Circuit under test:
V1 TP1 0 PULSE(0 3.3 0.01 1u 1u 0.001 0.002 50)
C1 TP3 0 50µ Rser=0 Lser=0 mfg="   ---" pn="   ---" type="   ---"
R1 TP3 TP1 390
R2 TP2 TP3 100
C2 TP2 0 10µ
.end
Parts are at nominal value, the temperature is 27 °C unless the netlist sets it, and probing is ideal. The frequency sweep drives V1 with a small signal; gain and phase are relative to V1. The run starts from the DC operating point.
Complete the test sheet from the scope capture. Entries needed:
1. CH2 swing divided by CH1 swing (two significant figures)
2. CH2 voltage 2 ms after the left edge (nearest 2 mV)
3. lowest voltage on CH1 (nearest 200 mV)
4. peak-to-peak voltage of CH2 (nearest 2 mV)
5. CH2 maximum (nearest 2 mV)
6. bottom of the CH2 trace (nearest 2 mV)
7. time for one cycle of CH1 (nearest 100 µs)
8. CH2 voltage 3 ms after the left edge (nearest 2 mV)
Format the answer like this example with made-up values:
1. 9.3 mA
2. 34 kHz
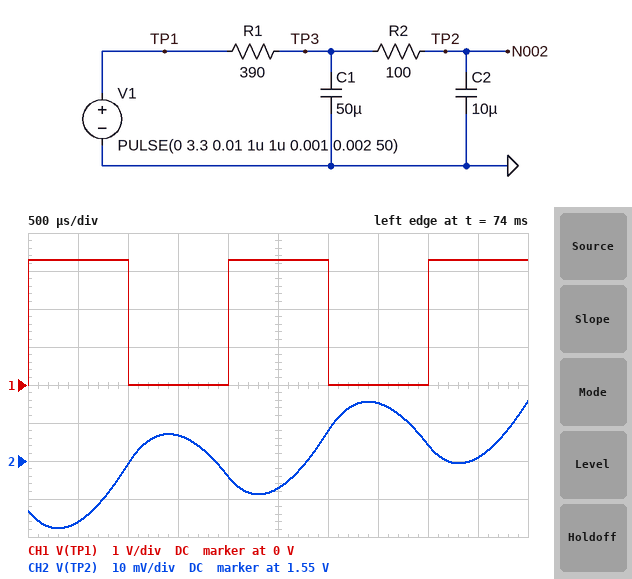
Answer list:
1. 0.010
2. 1.546 V
3. 0 V
4. 34 mV
5. 1.566 V
6. 1.532 V
7. 2.0 ms
8. 1.558 V
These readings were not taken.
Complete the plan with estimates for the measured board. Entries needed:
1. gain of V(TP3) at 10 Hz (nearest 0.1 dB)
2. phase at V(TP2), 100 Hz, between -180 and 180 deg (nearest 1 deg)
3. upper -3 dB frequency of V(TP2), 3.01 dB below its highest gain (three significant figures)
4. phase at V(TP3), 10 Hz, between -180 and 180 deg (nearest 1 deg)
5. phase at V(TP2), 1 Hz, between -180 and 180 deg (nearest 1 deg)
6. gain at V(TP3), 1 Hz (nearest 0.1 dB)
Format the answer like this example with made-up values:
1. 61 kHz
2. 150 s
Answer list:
1. -5.0 dB
2. -114 deg
3. 6.74 Hz
4. -55 deg
5. -9 deg
6. -0.1 dB
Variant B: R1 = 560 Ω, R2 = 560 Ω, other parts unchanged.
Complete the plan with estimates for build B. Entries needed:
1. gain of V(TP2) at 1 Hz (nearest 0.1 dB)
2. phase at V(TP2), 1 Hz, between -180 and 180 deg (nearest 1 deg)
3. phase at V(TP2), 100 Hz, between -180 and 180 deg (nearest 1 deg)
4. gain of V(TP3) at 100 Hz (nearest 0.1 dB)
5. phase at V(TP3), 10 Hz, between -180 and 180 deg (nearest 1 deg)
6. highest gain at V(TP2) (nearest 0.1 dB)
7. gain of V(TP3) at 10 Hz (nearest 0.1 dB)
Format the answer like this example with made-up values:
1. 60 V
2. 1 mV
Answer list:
1. -0.2 dB
2. -14 deg
3. -158 deg
4. -25.1 dB
5. -62 deg
6. 0 dB
7. -7.4 dB
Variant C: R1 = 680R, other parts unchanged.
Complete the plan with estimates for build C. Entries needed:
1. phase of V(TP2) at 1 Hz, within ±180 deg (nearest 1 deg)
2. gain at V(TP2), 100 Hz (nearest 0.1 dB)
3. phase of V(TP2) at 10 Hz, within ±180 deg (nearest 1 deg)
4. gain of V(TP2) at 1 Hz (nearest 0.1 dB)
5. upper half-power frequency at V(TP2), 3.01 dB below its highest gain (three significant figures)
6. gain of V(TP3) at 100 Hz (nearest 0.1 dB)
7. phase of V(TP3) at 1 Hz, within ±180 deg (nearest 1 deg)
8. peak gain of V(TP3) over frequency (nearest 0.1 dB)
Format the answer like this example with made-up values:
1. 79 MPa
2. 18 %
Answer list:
1. -15 deg
2. -29.3 dB
3. -72 deg
4. -0.3 dB
5. 3.88 Hz
6. -27.8 dB
7. -14 deg
8. 0 dB
